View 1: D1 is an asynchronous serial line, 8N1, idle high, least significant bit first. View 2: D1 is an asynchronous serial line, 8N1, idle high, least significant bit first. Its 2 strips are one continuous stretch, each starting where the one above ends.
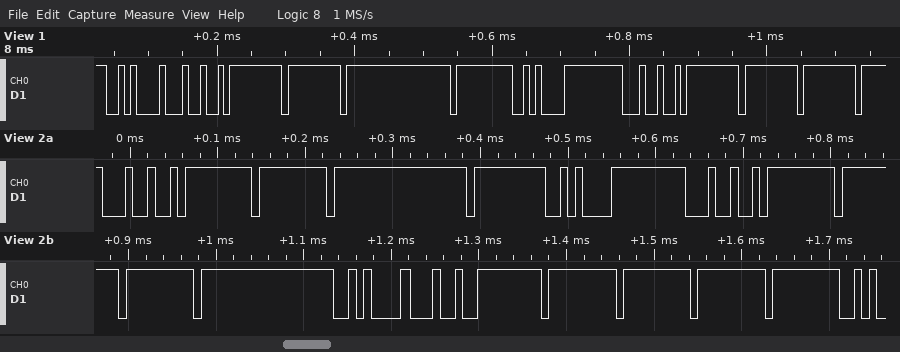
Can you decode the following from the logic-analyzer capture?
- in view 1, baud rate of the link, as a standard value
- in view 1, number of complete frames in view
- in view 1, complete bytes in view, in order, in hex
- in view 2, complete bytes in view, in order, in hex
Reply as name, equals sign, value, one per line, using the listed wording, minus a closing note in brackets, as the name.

in view 1, baud rate of the link, as a standard value = 115200 baud
in view 1, number of complete frames in view = 11
in view 1, complete bytes in view, in order, in hex = 0x0A 0x24 0xFF 0xFF 0xFF 0xFF 0x0A 0x24 0xFF 0xFF 0xFF
in view 2, complete bytes in view, in order, in hex = 24 FF FF FF FF 0A 24 FF FF FF FF 0A 24 FF FF FF FF
